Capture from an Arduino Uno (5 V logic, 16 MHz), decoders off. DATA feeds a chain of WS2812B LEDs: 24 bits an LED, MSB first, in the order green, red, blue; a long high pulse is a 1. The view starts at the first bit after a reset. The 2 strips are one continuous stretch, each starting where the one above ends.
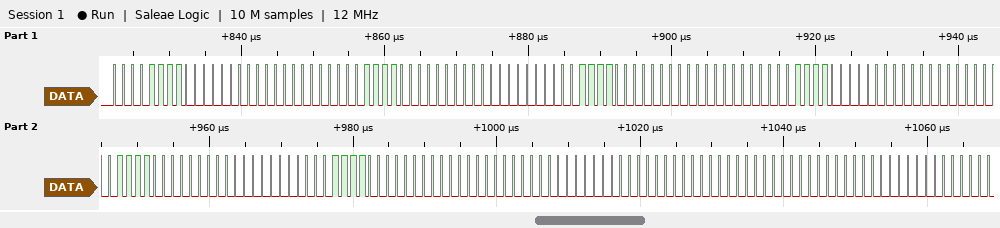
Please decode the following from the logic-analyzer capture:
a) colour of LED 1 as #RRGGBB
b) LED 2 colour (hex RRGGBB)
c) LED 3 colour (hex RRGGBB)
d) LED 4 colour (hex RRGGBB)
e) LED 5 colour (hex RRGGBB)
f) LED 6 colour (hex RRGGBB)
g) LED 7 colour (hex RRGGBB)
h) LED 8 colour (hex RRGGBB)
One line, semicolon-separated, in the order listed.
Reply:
#000F00; #000F00; #000F00; #000F00; #000F00; #000F00; #000000; #000000
